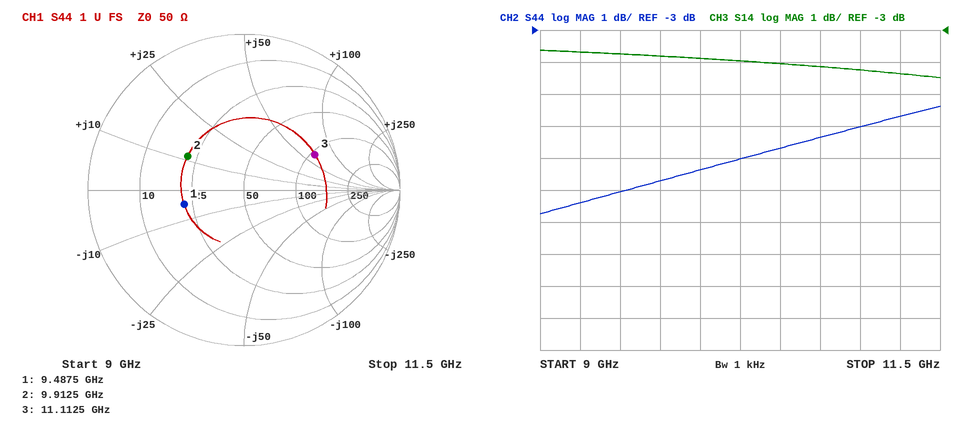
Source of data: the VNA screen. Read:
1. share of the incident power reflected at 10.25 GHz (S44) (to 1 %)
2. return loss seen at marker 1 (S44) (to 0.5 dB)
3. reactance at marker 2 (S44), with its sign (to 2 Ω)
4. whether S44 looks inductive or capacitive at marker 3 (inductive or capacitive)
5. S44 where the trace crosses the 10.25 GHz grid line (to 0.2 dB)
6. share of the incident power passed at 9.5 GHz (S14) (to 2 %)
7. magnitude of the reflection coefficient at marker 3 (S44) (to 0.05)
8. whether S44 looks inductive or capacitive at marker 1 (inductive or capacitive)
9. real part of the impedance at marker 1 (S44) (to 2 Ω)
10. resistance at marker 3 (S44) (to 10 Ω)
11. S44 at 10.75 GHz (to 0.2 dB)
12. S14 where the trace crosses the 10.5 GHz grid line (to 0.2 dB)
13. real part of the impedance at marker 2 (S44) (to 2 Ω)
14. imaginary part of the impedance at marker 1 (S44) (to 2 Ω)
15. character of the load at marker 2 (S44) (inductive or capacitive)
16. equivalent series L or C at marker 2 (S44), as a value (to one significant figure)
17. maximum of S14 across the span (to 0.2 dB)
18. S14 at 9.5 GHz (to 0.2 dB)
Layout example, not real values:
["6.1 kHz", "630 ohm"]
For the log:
["20 %", "8.0 dB", "+12 Ω", "inductive", "-7.0 dB", "42 %", "0.50", "capacitive", "22 Ω", "110 Ω", "-6.4 dB", "-4.0 dB", "22 Ω", "-4 Ω", "inductive", "200 pH", "-3.6 dB", "-3.8 dB"]
